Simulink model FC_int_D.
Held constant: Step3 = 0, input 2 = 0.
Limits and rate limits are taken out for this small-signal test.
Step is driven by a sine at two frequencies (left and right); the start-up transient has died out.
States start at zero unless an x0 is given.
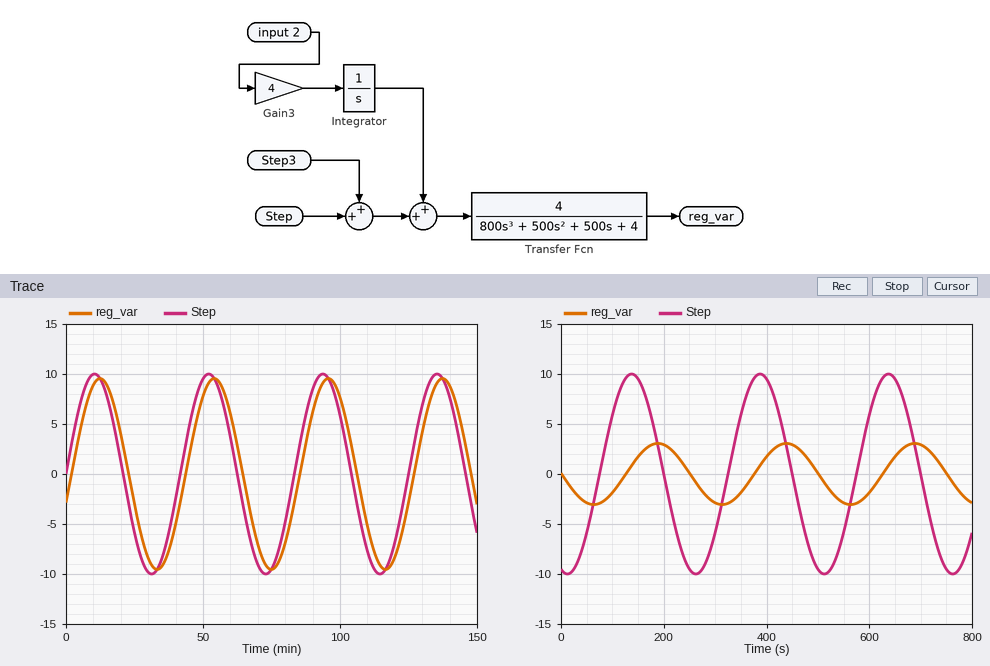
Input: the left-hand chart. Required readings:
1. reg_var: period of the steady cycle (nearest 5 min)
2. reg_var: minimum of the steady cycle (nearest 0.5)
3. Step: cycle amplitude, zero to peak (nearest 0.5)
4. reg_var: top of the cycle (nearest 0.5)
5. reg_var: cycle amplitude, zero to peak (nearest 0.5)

40 min
-9.5
10.0
9.5
9.5
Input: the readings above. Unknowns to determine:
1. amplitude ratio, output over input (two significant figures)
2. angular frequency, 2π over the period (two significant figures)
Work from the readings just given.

0.95
0.16 rad/min
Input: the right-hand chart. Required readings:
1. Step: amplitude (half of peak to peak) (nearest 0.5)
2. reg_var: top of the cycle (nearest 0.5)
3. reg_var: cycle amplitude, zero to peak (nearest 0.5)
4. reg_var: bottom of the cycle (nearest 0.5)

10.0
3.0
3.0
-3.0
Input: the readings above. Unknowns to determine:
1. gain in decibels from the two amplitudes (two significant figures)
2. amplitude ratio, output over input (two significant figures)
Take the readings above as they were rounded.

-10 dB
0.30
